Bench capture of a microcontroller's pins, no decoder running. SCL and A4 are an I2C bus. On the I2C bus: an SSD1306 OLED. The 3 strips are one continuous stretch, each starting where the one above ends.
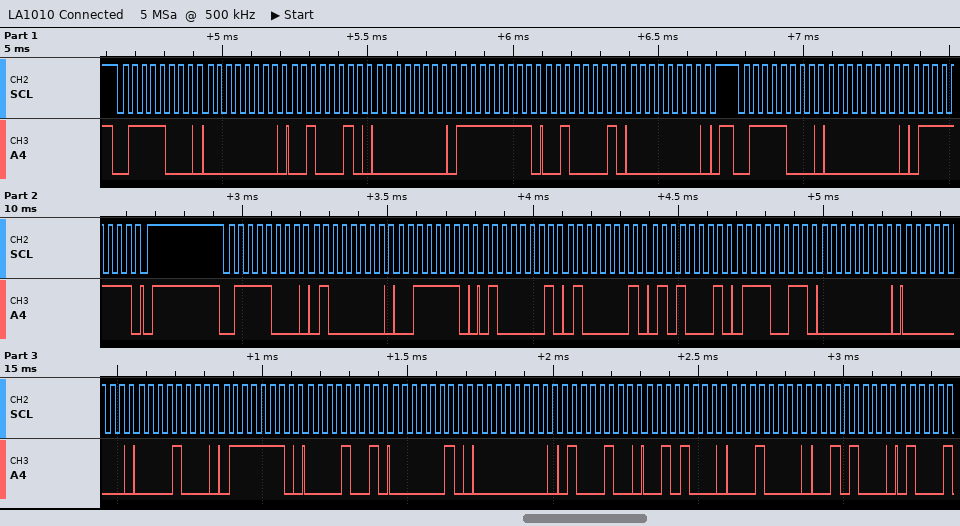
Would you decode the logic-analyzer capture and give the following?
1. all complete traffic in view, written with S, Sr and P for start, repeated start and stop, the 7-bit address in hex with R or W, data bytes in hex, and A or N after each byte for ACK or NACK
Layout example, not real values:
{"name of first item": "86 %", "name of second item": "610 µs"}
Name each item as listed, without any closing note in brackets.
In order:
{"all complete traffic in view, written with S, Sr and P for start, repeated start and stop, the 7-bit address in hex with R or W, data bytes in hex, and A or N after each byte for ACK or NACK": "S 3CW A 00 A 22 A 00 A FF A 21 A 00 A P S 3CW A 00 A 7F A P S 3CW A 40 A 3E A 41 A 41 A 51 A 73 A 00 A 00 A 08 A 7E A 09 A 02 A 00 A 44 A 28 A 10 A 28 A"}
